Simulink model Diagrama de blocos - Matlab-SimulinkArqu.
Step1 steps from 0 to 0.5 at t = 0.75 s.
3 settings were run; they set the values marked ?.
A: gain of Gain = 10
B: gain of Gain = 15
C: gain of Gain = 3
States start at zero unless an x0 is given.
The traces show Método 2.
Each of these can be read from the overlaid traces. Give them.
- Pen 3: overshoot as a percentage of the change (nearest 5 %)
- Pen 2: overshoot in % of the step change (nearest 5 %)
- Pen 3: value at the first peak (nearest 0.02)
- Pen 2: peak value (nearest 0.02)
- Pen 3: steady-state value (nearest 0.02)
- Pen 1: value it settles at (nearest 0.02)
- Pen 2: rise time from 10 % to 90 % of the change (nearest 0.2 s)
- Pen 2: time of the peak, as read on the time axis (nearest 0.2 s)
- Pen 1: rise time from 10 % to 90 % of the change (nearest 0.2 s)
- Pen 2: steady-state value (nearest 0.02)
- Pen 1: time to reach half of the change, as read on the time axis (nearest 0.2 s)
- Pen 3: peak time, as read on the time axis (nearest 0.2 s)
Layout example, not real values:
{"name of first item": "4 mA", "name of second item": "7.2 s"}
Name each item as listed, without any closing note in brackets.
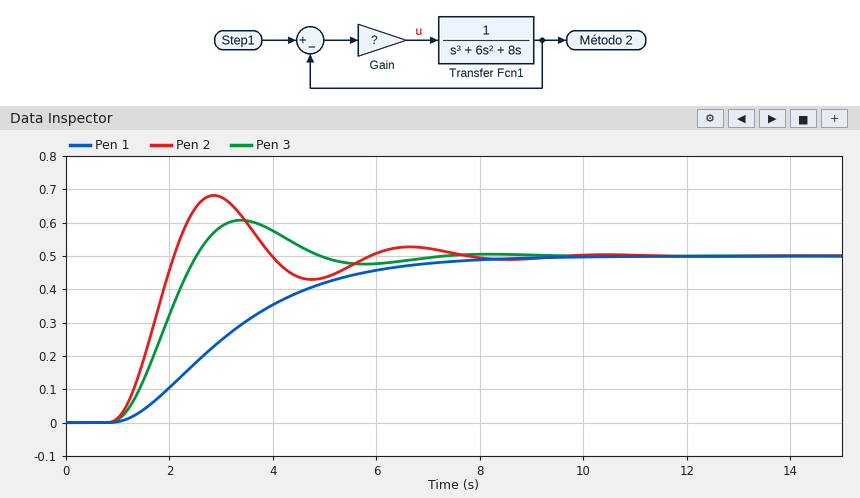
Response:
{"Pen 3: overshoot as a percentage of the change": "20 %", "Pen 2: overshoot in % of the step change": "35 %", "Pen 3: value at the first peak": "0.60", "Pen 2: peak value": "0.68", "Pen 3: steady-state value": "0.50", "Pen 1: value it settles at": "0.50", "Pen 2: rise time from 10 % to 90 % of the change": "0.8 s", "Pen 2: time of the peak, as read on the time axis": "2.8 s", "Pen 1: rise time from 10 % to 90 % of the change": "4.2 s", "Pen 2: steady-state value": "0.50", "Pen 1: time to reach half of the change, as read on the time axis": "3.0 s", "Pen 3: peak time, as read on the time axis": "3.4 s"}
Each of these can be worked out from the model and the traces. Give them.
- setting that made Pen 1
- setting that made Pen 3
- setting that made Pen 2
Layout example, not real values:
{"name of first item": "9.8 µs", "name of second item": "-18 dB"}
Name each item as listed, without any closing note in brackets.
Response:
{"setting that made Pen 1": "C", "setting that made Pen 3": "A", "setting that made Pen 2": "B"}
